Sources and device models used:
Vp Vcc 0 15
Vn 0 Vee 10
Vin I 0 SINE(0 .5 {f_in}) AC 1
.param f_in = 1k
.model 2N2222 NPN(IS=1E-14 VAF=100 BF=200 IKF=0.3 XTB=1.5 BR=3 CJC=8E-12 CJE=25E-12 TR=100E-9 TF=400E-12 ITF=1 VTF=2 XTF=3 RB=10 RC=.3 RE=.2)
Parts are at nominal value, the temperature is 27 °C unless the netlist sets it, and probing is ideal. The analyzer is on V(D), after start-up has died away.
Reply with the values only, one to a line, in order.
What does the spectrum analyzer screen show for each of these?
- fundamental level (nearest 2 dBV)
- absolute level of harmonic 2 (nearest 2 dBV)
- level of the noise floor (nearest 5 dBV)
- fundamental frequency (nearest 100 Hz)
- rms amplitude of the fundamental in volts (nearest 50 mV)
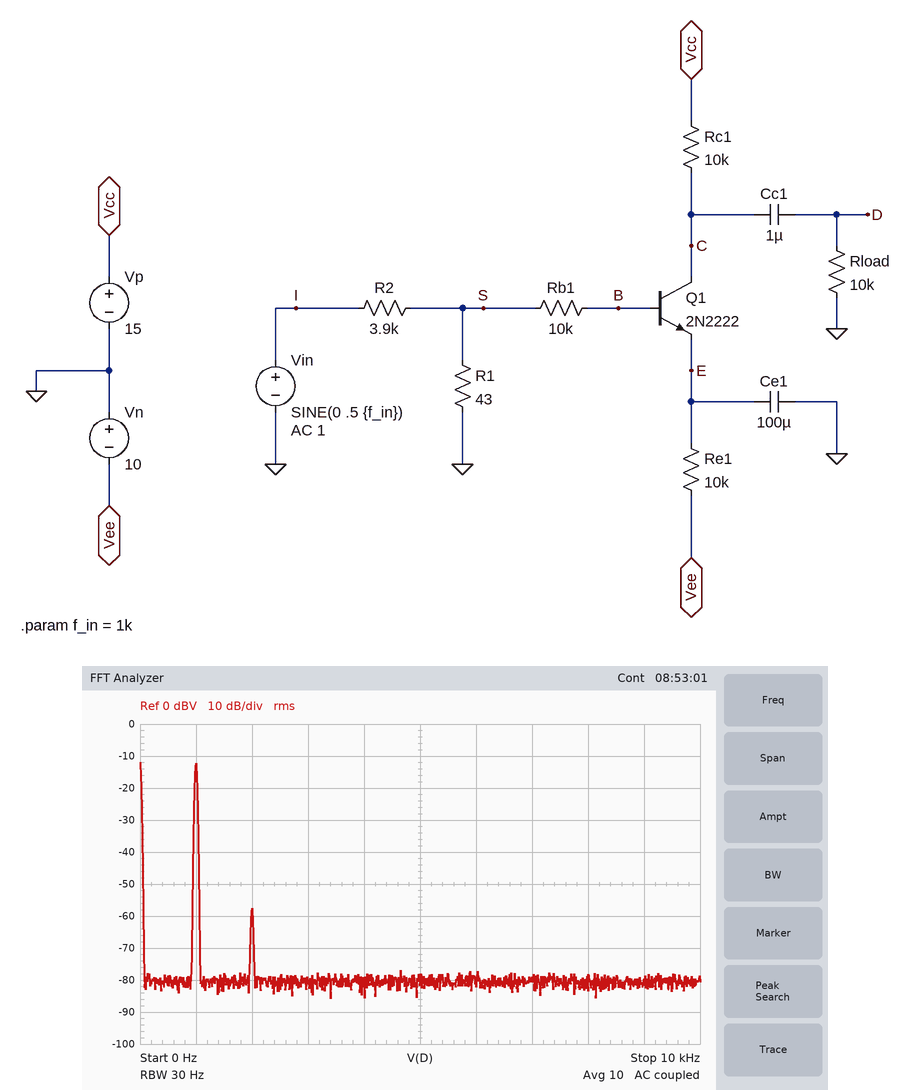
-12 dBV
-58 dBV
-80 dBV
1.0 kHz
250 mV
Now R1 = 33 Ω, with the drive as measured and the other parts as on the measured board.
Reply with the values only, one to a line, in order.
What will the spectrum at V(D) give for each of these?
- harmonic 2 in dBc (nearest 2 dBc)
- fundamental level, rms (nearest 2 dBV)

-48 dBc
-14 dBV
